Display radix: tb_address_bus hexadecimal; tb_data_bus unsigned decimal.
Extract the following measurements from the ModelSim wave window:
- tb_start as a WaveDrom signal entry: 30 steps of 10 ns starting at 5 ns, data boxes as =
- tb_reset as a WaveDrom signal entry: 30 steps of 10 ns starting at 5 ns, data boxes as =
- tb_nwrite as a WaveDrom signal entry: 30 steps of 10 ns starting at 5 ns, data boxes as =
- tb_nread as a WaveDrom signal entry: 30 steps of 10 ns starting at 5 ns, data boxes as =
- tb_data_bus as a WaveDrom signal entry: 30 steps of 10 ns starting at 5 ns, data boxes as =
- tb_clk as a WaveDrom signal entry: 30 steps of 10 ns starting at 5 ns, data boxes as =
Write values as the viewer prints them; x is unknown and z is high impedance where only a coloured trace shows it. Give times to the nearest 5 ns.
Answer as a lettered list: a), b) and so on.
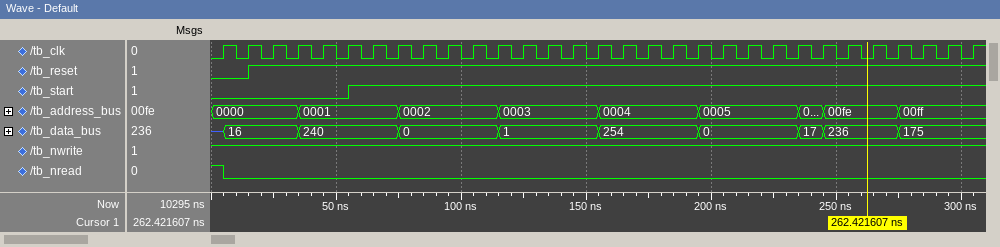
a) {name: 'tb_start', wave: '0....1........................'}
b) {name: 'tb_reset', wave: '01............................'}
c) {name: 'tb_nwrite', wave: '1.............................'}
d) {name: 'tb_nread', wave: '0.............................'}
e) {name: 'tb_data_bus', wave: '=..=...=...=...=...=...==..=..', data: '16 240 0 1 254 0 17 236 175'}
f) {name: 'tb_clk', wave: 'p.............................'}
